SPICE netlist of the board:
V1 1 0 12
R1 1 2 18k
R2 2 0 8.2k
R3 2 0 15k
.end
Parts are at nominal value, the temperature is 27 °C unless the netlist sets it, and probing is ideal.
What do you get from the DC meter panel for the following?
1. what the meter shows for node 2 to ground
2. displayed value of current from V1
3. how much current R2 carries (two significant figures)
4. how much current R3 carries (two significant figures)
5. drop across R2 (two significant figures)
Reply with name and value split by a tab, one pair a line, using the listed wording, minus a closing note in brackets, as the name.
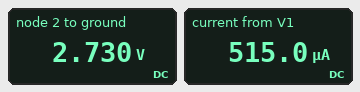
what the meter shows for node 2 to ground	2.730 V
displayed value of current from V1	515.0 µA
how much current R2 carries	330 µA
how much current R3 carries	180 µA
drop across R2	2.7 V
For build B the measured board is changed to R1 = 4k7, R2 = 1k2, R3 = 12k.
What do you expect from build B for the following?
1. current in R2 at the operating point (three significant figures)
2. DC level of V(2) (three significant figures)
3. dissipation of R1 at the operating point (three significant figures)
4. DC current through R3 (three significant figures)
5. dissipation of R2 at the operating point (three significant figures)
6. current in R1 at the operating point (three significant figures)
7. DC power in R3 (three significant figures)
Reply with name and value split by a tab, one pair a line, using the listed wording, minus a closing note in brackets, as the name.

current in R2 at the operating point	1.88 mA
DC level of V(2)	2.26 V
dissipation of R1 at the operating point	20.2 mW
DC current through R3	188 µA
dissipation of R2 at the operating point	4.26 mW
current in R1 at the operating point	2.07 mA
DC power in R3	426 µW
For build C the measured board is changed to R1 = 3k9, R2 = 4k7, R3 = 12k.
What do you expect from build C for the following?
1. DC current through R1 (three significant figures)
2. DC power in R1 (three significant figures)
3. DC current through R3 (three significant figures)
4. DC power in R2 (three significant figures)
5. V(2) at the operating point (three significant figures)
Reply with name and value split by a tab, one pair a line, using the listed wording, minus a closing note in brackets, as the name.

DC current through R1	1.65 mA
DC power in R1	10.6 mW
DC current through R3	464 µA
DC power in R2	6.60 mW
V(2) at the operating point	5.57 V
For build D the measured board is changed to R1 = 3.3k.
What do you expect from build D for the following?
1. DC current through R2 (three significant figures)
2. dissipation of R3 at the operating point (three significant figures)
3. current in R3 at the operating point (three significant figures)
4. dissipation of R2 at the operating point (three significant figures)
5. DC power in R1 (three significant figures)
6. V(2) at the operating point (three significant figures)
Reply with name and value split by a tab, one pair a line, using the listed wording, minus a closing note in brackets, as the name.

DC current through R2	902 µA
dissipation of R3 at the operating point	3.65 mW
current in R3 at the operating point	493 µA
dissipation of R2 at the operating point	6.67 mW
DC power in R1	6.42 mW
V(2) at the operating point	7.40 V
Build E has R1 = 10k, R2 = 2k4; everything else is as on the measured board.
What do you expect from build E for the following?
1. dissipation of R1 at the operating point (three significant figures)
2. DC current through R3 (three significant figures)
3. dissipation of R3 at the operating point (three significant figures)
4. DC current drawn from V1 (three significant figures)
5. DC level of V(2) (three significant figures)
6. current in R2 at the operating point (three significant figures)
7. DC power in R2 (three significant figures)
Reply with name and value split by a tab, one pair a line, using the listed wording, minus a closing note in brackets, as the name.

dissipation of R1 at the operating point	9.89 mW
DC current through R3	137 µA
dissipation of R3 at the operating point	282 µW
DC current drawn from V1	994 µA
DC level of V(2)	2.06 V
current in R2 at the operating point	857 µA
DC power in R2	1.76 mW
